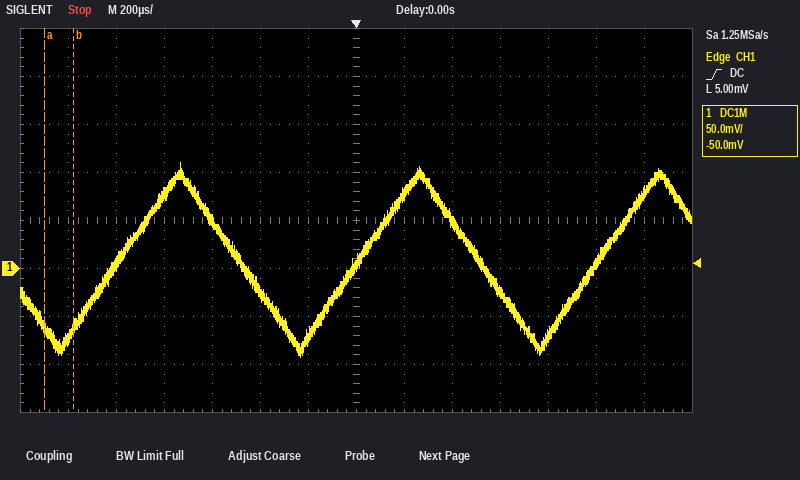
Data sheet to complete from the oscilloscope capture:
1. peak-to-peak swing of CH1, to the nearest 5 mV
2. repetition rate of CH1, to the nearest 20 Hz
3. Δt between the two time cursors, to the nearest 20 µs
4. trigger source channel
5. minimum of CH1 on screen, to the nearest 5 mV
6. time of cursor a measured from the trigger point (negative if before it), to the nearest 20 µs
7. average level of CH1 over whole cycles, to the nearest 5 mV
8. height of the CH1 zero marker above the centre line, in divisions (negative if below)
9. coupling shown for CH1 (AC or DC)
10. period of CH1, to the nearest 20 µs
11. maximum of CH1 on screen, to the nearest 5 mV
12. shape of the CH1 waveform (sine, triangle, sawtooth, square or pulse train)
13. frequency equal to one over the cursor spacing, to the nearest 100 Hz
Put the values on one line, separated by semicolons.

200 mV; 1.00 kHz; 120 µs; CH1; -90 mV; -1.30 ms; 10 mV; -1.0 div; DC; 1.00 ms; 110 mV; triangle; 8.3 kHz
